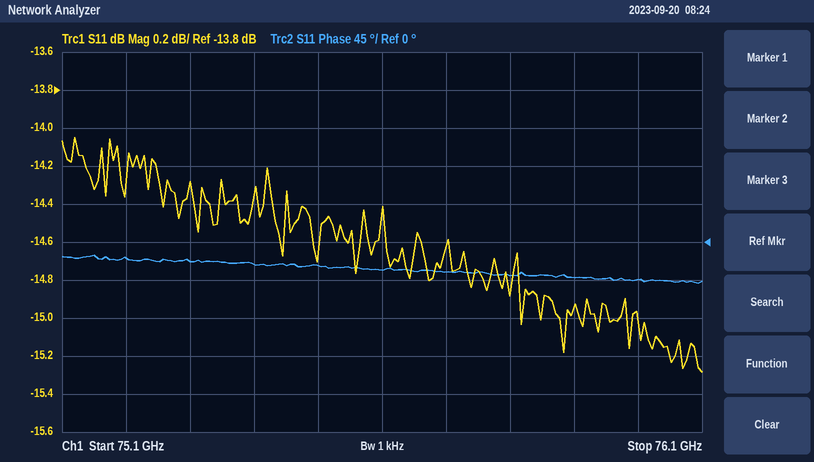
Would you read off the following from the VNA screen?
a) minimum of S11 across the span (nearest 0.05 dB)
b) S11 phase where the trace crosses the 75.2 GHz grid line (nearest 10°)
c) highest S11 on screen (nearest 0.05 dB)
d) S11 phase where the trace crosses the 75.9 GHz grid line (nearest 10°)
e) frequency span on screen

-15.30 dB
-20°
-14.05 dB
-40°
1 GHz
